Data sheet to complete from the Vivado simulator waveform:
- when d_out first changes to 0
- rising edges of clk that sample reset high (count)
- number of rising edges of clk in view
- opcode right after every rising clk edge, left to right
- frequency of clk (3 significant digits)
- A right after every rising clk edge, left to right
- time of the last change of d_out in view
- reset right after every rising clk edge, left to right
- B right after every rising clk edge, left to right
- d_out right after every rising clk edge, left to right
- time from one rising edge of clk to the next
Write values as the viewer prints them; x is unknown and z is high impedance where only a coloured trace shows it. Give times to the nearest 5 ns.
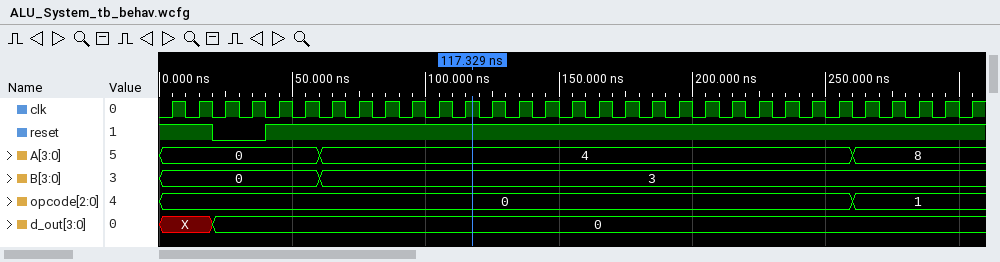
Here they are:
20 ns
29
31
0, 0, 0, 0, 0, 0, 0, 0, 0, 0, 0, 0, 0, 0, 0, 0, 0, 0, 0, 0, 0, 0, 0, 0, 0, 0, 1, 1, 1, 1, 1
100 MHz
0, 0, 0, 0, 0, 0, 4, 4, 4, 4, 4, 4, 4, 4, 4, 4, 4, 4, 4, 4, 4, 4, 4, 4, 4, 4, 8, 8, 8, 8, 8
20 ns
1 1 0 0 1 1 1 1 1 1 1 1 1 1 1 1 1 1 1 1 1 1 1 1 1 1 1 1 1 1 1
0, 0, 0, 0, 0, 0, 3, 3, 3, 3, 3, 3, 3, 3, 3, 3, 3, 3, 3, 3, 3, 3, 3, 3, 3, 3, 3, 3, 3, 3, 3
X, X, 0, 0, 0, 0, 0, 0, 0, 0, 0, 0, 0, 0, 0, 0, 0, 0, 0, 0, 0, 0, 0, 0, 0, 0, 0, 0, 0, 0, 0
10 ns
